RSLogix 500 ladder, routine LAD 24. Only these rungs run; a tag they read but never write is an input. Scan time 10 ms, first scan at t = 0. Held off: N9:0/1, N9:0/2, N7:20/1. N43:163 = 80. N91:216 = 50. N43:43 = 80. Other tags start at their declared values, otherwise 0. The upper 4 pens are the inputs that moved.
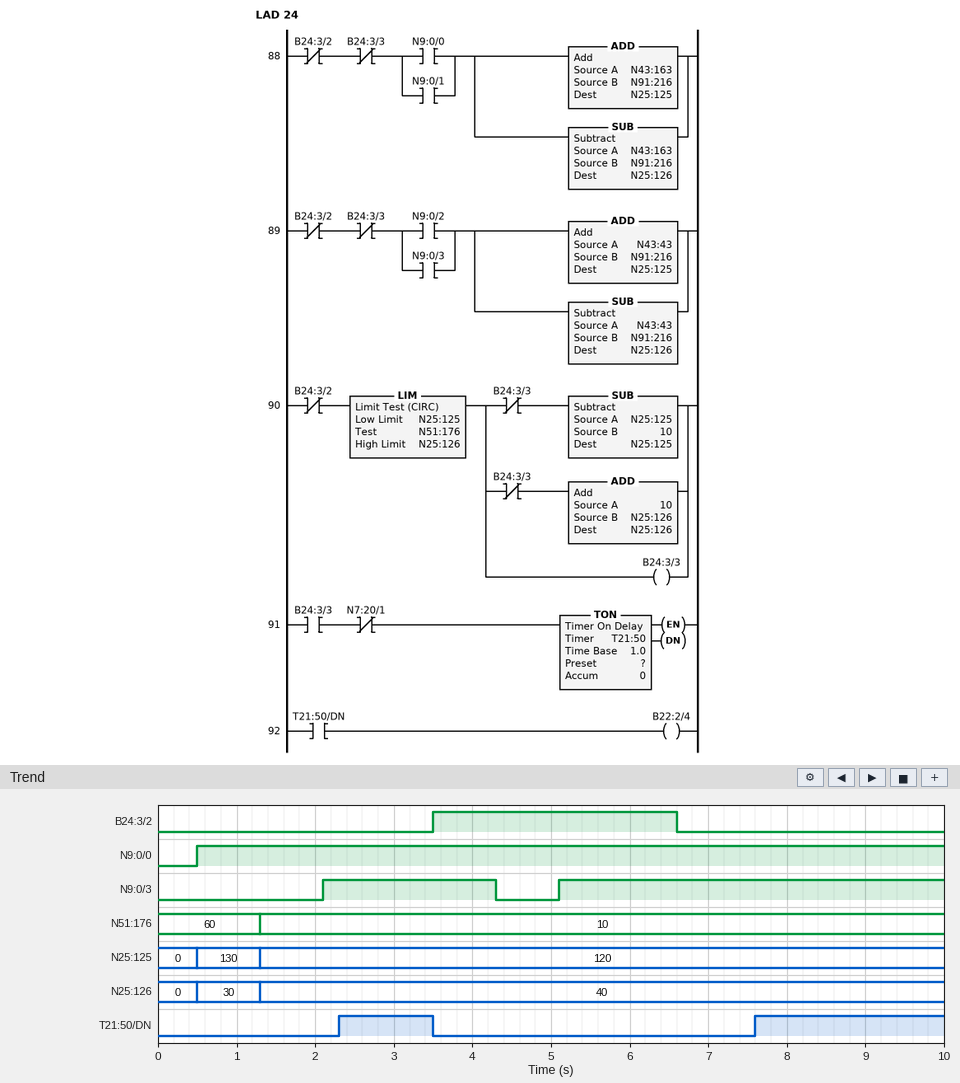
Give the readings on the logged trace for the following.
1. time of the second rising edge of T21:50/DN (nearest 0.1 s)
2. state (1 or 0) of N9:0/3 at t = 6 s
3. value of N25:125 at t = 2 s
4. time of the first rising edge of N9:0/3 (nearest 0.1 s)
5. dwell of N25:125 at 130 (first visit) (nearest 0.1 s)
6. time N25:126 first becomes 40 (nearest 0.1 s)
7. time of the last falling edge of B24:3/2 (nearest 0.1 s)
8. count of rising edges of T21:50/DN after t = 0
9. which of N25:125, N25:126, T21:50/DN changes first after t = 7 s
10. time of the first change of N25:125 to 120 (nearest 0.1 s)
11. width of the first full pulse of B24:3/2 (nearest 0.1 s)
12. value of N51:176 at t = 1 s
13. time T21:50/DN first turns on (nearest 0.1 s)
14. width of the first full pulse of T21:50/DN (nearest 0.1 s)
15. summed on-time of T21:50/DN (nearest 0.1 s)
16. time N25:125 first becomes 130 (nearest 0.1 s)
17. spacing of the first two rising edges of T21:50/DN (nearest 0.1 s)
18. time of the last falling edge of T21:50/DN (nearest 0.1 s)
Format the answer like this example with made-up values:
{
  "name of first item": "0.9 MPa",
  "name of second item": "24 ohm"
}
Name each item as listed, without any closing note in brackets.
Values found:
{
  "time of the second rising edge of T21:50/DN": "7.6 s",
  "state (1 or 0) of N9:0/3 at t = 6 s": "1",
  "value of N25:125 at t = 2 s": "120",
  "time of the first rising edge of N9:0/3": "2.1 s",
  "dwell of N25:125 at 130 (first visit)": "0.8 s",
  "time N25:126 first becomes 40": "1.3 s",
  "time of the last falling edge of B24:3/2": "6.6 s",
  "count of rising edges of T21:50/DN after t = 0": "2",
  "which of N25:125, N25:126, T21:50/DN changes first after t = 7 s": "T21:50/DN",
  "time of the first change of N25:125 to 120": "1.3 s",
  "width of the first full pulse of B24:3/2": "3.1 s",
  "value of N51:176 at t = 1 s": "60",
  "time T21:50/DN first turns on": "2.3 s",
  "width of the first full pulse of T21:50/DN": "1.2 s",
  "summed on-time of T21:50/DN": "3.6 s",
  "time N25:125 first becomes 130": "0.5 s",
  "spacing of the first two rising edges of T21:50/DN": "5.3 s",
  "time of the last falling edge of T21:50/DN": "3.5 s"
}
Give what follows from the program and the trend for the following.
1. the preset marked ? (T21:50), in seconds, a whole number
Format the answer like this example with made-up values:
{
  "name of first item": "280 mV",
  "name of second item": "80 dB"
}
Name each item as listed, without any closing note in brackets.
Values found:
{
  "the preset marked ? (T21:50), in seconds, a whole number": "1 s"
}
